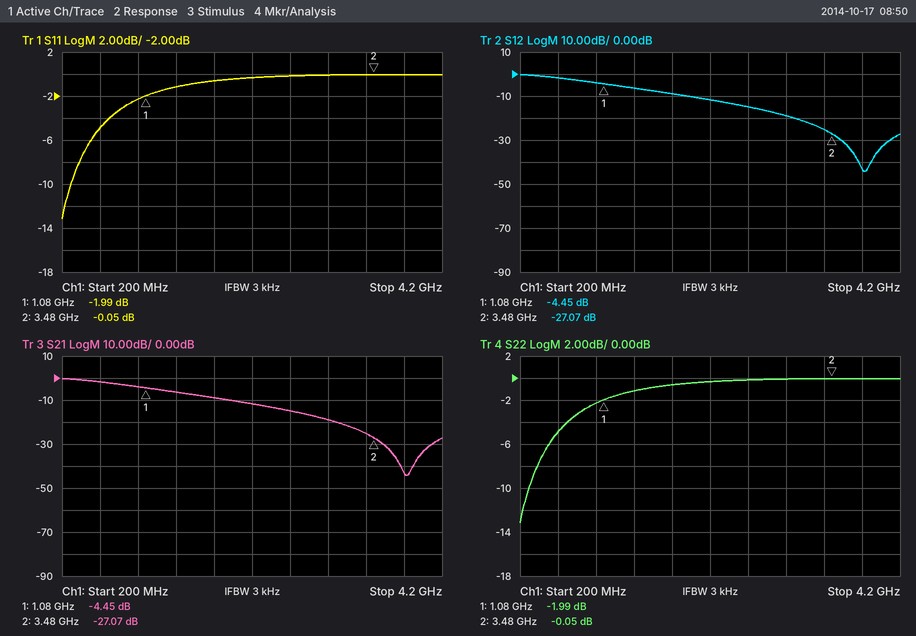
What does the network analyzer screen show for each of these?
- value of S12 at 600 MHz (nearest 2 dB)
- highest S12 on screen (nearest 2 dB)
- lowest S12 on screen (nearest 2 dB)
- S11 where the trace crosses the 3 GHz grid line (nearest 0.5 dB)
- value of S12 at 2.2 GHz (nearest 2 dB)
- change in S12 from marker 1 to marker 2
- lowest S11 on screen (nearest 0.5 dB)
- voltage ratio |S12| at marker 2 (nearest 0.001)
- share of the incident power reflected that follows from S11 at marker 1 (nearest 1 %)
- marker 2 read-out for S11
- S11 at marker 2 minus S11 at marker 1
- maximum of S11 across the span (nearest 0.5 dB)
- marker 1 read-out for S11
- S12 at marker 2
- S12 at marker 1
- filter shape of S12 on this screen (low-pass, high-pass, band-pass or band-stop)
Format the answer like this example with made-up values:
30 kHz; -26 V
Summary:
-2 dB; 0 dB; -44 dB; 0.0 dB; -12 dB; -22.62 dB; -13.0 dB; 0.044; 63 %; -0.05 dB; 1.94 dB; 0.0 dB; -1.99 dB; -27.07 dB; -4.45 dB; low-pass
